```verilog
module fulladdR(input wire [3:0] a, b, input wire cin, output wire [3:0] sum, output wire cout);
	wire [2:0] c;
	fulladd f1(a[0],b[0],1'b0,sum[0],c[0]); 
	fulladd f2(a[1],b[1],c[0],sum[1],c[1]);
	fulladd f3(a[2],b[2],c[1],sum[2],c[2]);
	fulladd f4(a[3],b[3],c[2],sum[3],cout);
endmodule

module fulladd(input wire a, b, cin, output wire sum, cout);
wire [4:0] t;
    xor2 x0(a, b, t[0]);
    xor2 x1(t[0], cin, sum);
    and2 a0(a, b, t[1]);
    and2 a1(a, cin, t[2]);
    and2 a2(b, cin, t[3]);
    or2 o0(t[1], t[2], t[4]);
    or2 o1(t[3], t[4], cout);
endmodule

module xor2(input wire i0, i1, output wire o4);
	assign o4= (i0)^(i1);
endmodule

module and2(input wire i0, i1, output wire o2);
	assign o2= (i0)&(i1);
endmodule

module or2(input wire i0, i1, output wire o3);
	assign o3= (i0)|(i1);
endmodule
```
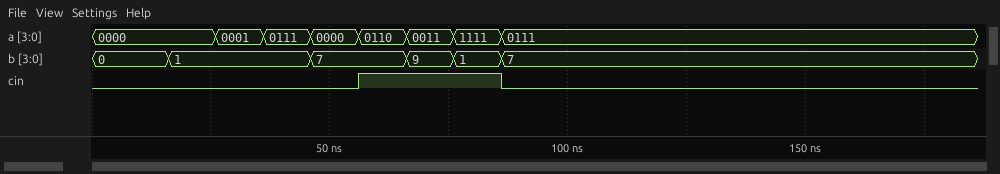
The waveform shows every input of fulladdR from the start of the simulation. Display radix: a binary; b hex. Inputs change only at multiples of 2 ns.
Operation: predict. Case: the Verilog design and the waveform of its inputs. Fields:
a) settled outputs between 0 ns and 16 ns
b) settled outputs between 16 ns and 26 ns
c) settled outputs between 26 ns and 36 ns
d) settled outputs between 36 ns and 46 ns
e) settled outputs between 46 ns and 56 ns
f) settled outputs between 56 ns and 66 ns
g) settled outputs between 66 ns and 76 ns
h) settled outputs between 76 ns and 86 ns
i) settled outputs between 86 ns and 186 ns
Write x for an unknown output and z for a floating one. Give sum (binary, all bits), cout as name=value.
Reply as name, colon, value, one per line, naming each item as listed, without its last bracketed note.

settled outputs between 0 ns and 16 ns: sum=0000, cout=0
settled outputs between 16 ns and 26 ns: sum=0001, cout=0
settled outputs between 26 ns and 36 ns: sum=0010, cout=0
settled outputs between 36 ns and 46 ns: sum=1000, cout=0
settled outputs between 46 ns and 56 ns: sum=0111, cout=0
settled outputs between 56 ns and 66 ns: sum=1101, cout=0
settled outputs between 66 ns and 76 ns: sum=1100, cout=0
settled outputs between 76 ns and 86 ns: sum=0000, cout=1
settled outputs between 86 ns and 186 ns: sum=1110, cout=0
